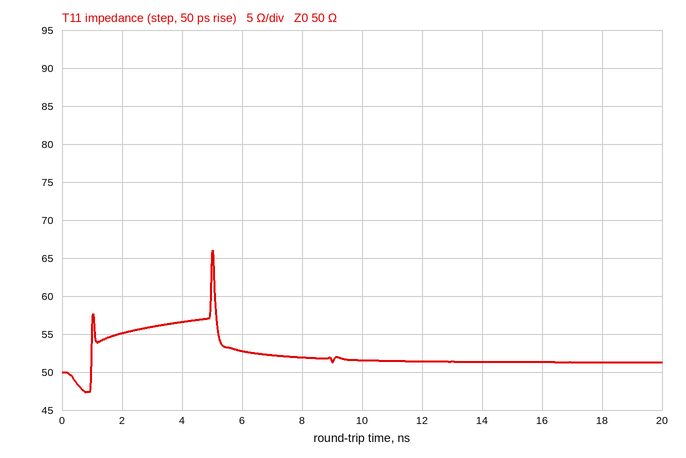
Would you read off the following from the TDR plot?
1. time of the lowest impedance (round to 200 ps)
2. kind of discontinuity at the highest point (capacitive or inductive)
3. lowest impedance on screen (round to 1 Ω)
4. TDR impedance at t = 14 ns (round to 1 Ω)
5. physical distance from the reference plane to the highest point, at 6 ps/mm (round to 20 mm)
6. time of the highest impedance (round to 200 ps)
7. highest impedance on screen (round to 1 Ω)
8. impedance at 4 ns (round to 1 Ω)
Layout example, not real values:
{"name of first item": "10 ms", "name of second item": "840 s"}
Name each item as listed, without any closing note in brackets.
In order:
{"time of the lowest impedance": "800 ps", "kind of discontinuity at the highest point": "inductive", "lowest impedance on screen": "47 Ω", "TDR impedance at t = 14 ns": "51 Ω", "physical distance from the reference plane to the highest point, at 6 ps/mm": "420 mm", "time of the highest impedance": "5.0 ns", "highest impedance on screen": "66 Ω", "impedance at 4 ns": "57 Ω"}
